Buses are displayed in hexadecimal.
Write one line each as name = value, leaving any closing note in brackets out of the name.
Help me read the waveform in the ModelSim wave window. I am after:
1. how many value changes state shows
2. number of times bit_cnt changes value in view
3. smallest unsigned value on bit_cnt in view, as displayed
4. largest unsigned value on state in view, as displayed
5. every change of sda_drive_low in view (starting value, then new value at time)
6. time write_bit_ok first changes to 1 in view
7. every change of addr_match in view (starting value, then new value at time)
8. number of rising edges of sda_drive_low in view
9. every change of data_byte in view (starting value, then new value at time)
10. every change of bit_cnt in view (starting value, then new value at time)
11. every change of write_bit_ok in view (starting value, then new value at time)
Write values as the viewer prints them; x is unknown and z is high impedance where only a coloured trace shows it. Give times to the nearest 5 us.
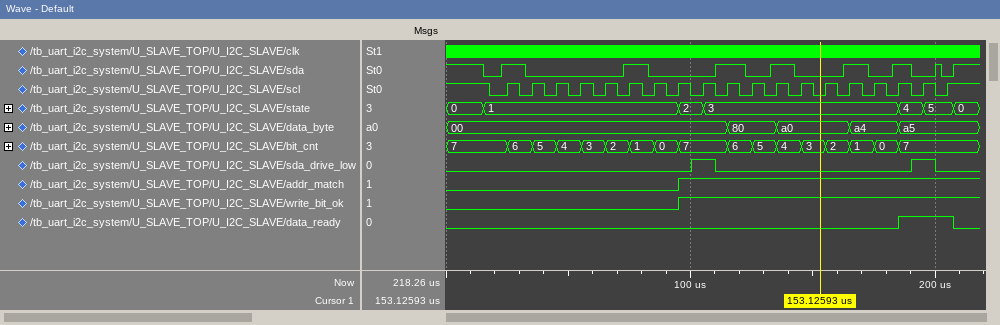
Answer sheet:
how many value changes state shows = 6
number of times bit_cnt changes value in view = 16
smallest unsigned value on bit_cnt in view, as displayed = 0
largest unsigned value on state in view, as displayed = 5
every change of sda_drive_low in view = 0, 1 at 100 us, 0 at 110 us, 1 at 190 us, 0 at 200 us
time write_bit_ok first changes to 1 in view = 95 us
every change of addr_match in view = 0, 1 at 95 us
number of rising edges of sda_drive_low in view = 2
every change of data_byte in view = 00, 80 at 115 us, a0 at 135 us, a4 at 165 us, a5 at 185 us
every change of bit_cnt in view = 7, 6 at 25 us, 5 at 35 us, 4 at 45 us, 3 at 55 us, 2 at 65 us, 1 at 75 us, 0 at 85 us, 7 at 95 us, 6 at 115 us, 5 at 125 us, 4 at 135 us, 3 at 145 us, 2 at 155 us, 1 at 165 us, 0 at 175 us, 7 at 185 us
every change of write_bit_ok in view = 0, 1 at 95 us
